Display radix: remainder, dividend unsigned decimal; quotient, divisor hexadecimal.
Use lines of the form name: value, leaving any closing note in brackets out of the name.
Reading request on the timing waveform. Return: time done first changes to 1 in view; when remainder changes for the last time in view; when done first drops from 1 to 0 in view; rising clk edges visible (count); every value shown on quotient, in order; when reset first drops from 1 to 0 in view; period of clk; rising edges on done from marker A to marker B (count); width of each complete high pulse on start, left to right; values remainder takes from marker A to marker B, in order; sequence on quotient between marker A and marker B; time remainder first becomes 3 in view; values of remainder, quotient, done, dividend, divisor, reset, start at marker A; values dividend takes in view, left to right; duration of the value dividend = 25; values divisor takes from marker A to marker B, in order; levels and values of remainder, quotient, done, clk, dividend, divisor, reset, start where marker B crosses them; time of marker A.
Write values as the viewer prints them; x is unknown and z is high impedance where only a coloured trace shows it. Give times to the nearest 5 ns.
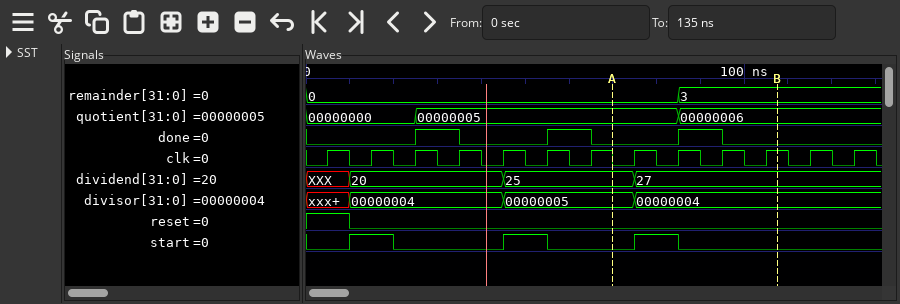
time done first changes to 1 in view: 25 ns
when remainder changes for the last time in view: 85 ns
when done first drops from 1 to 0 in view: 35 ns
rising clk edges visible: 13
every value shown on quotient, in order: 00000000, 00000005, 00000006
when reset first drops from 1 to 0 in view: 10 ns
period of clk: 10 ns
rising edges on done from marker A to marker B: 1
width of each complete high pulse on start, left to right: 10 ns, 10 ns, 10 ns
values remainder takes from marker A to marker B, in order: 0, 3
sequence on quotient between marker A and marker B: 00000005, 00000006
time remainder first becomes 3 in view: 85 ns
values of remainder, quotient, done, dividend, divisor, reset, start at marker A: remainder=0, quotient=00000005, done=0, dividend=25, divisor=00000005, reset=0, start=0
values dividend takes in view, left to right: XXX, 20, 25, 27
duration of the value dividend = 25: 30 ns
values divisor takes from marker A to marker B, in order: 00000005, 00000004
levels and values of remainder, quotient, done, clk, dividend, divisor, reset, start where marker B crosses them: remainder=3, quotient=00000006, done=0, clk=1, dividend=27, divisor=00000004, reset=0, start=0
time of marker A: 70 ns
